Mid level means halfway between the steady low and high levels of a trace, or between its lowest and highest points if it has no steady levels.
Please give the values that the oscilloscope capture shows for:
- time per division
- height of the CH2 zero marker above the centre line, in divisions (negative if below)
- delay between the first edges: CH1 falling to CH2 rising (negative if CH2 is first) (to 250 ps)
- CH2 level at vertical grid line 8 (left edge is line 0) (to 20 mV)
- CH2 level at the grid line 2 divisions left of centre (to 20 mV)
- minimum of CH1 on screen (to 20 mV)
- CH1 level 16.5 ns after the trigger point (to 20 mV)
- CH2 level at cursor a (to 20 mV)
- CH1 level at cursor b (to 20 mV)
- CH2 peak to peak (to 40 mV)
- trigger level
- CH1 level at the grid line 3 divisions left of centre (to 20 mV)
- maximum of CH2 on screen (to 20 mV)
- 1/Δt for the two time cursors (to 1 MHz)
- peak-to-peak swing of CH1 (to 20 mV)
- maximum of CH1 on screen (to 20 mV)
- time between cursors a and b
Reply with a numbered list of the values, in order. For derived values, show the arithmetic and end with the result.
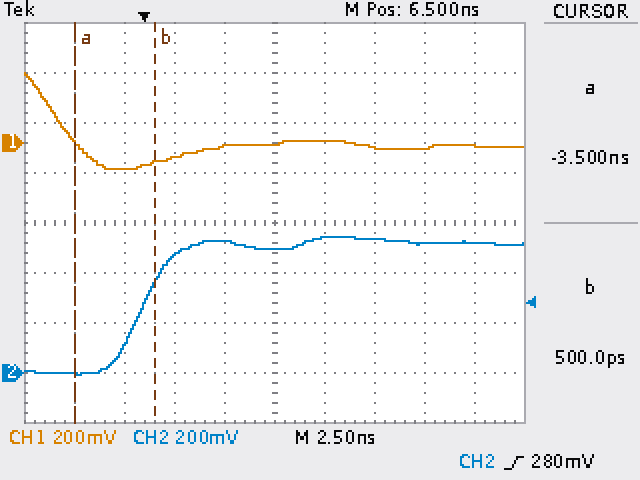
1. 2.5 ns
2. -3.0 div
3. +4.25 ns
4. 520 mV
5. 460 mV
6. -100 mV
7. -20 mV
8. 0 mV
9. -80 mV
10. 560 mV
11. 280 mV
12. -100 mV
13. 540 mV
14. 1 / 4.00 ns ≈ 250 MHz
15. 280 mV − (-100 mV) = 380 mV
16. 280 mV
17. 500 ps − (-3.5 ns) = 4.00 ns
